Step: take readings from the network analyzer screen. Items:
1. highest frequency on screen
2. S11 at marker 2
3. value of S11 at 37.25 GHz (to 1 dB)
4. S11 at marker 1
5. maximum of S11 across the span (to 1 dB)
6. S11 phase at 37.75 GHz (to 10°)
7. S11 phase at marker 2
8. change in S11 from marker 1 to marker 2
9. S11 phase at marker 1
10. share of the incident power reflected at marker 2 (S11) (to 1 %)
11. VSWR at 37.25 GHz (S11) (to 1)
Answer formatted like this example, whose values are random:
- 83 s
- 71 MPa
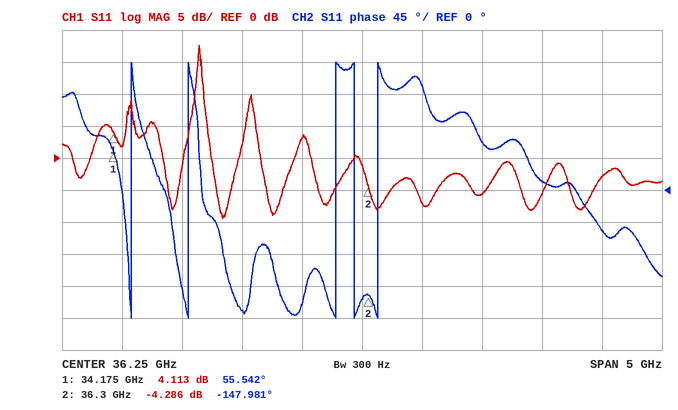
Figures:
- 38.75 GHz
- -4.286 dB
- -6 dB
- 4.113 dB
- 18 dB
- 10°
- -147.981°
- -8.399 dB
- 55.542°
- 37 %
- 3
